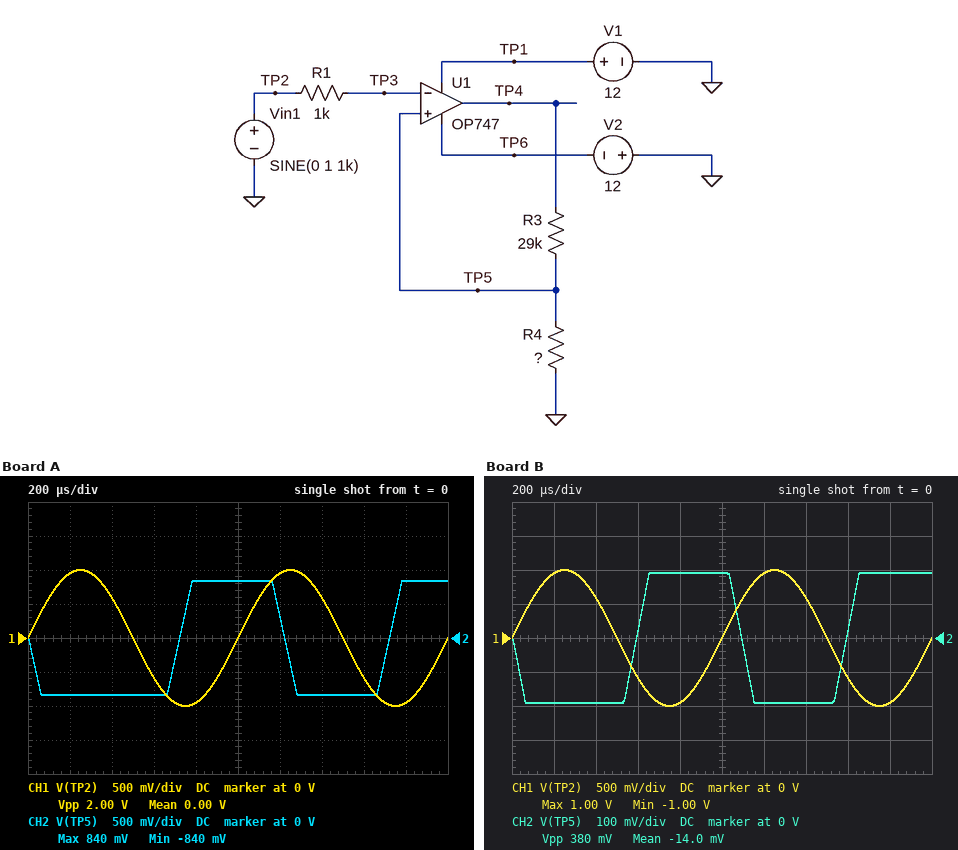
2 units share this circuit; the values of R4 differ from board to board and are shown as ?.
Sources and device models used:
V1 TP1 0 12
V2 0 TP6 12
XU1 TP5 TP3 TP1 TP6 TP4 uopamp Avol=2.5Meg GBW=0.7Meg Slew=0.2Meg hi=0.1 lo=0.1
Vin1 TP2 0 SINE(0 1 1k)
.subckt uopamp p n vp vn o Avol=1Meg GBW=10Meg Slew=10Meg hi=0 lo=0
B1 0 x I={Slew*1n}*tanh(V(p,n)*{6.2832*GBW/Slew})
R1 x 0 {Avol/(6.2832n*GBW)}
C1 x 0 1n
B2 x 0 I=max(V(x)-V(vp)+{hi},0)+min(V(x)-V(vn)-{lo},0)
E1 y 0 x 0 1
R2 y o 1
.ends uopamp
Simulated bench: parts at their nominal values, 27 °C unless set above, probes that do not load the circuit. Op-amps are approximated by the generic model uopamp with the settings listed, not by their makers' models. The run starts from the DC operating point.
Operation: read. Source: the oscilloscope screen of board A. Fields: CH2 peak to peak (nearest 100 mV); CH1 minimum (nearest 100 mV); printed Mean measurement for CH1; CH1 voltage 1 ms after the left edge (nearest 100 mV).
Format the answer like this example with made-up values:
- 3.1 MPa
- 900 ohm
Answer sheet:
- 1.7 V
- -1.0 V
- 0.00 V
- 0 V
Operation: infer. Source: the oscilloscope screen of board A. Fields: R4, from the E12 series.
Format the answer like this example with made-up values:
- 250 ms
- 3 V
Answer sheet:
- 2.2 kΩ
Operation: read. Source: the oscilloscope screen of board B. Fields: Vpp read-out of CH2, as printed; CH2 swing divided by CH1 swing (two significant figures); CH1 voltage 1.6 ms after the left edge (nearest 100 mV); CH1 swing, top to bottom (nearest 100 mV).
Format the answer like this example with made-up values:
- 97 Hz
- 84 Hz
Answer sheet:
- 380 mV
- 0.19
- -600 mV
- 2.0 V
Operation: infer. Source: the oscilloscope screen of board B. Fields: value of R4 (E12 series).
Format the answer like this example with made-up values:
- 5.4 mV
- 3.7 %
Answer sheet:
- 470 Ω
